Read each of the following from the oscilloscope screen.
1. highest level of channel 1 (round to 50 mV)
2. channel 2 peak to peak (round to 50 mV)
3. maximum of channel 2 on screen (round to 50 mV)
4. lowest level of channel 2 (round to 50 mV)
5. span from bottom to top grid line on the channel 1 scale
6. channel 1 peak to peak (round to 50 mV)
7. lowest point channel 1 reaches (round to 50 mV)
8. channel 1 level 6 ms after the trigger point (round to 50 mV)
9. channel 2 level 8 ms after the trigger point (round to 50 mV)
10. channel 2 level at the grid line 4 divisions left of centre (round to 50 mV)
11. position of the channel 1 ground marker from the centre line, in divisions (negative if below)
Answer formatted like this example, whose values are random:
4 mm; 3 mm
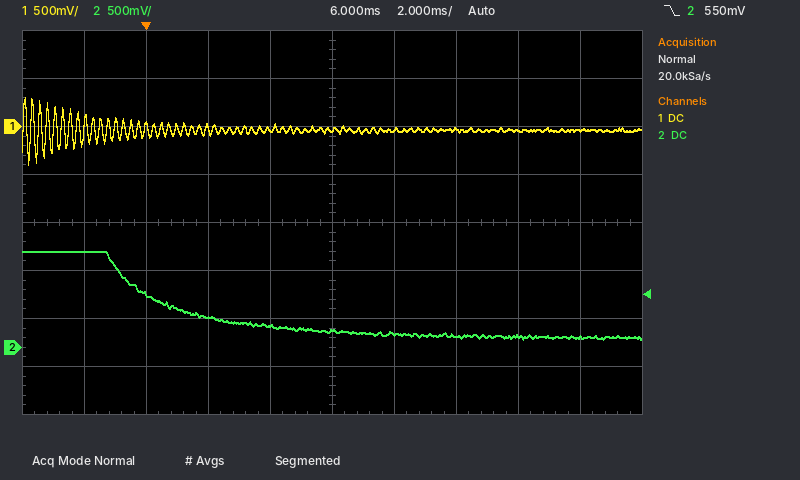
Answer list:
300 mV; 900 mV; 1.00 V; 100 mV; 4 V; 700 mV; -400 mV; -50 mV; 150 mV; 1.00 V; +2.0 div
